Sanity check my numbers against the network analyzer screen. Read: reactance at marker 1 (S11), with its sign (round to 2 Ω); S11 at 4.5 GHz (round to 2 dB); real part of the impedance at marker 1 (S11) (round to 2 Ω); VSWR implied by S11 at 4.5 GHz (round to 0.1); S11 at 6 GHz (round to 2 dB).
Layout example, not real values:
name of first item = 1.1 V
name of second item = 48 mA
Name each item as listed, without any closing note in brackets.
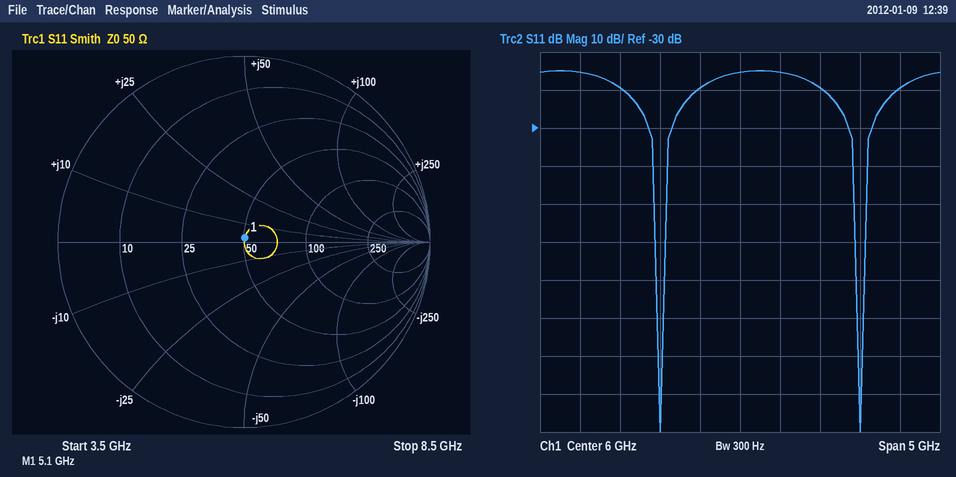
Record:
reactance at marker 1 (S11), with its sign = +2 Ω
S11 at 4.5 GHz = -20 dB
real part of the impedance at marker 1 (S11) = 50 Ω
VSWR implied by S11 at 4.5 GHz = 1.2
S11 at 6 GHz = -16 dB
